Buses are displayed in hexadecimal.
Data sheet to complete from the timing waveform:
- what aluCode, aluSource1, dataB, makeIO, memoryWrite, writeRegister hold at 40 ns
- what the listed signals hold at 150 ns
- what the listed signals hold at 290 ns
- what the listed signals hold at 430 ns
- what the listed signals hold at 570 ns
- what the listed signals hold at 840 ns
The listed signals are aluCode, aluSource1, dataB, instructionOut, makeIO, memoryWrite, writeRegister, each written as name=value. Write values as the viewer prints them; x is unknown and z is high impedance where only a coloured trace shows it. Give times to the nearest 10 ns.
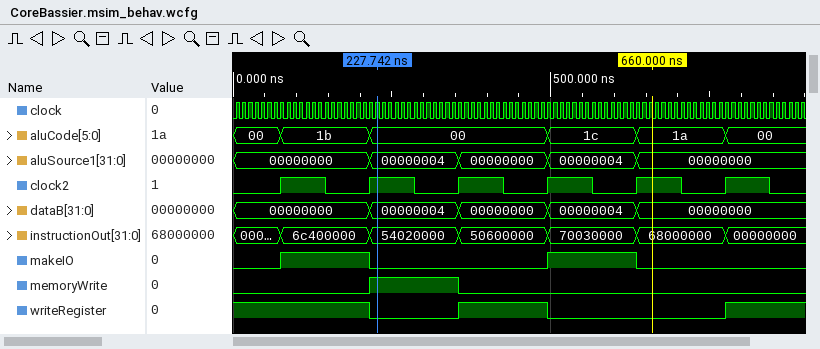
aluCode=00, aluSource1=00000000, dataB=00000000, makeIO=0, memoryWrite=0, writeRegister=1
aluCode=1b, aluSource1=00000000, dataB=00000000, instructionOut=6c400000, makeIO=1, memoryWrite=0, writeRegister=1
aluCode=00, aluSource1=00000004, dataB=00000004, instructionOut=54020000, makeIO=0, memoryWrite=1, writeRegister=0
aluCode=00, aluSource1=00000000, dataB=00000000, instructionOut=50600000, makeIO=0, memoryWrite=0, writeRegister=1
aluCode=1c, aluSource1=00000004, dataB=00000004, instructionOut=70030000, makeIO=1, memoryWrite=0, writeRegister=0
aluCode=00, aluSource1=00000000, dataB=00000000, instructionOut=00000000, makeIO=0, memoryWrite=0, writeRegister=1
